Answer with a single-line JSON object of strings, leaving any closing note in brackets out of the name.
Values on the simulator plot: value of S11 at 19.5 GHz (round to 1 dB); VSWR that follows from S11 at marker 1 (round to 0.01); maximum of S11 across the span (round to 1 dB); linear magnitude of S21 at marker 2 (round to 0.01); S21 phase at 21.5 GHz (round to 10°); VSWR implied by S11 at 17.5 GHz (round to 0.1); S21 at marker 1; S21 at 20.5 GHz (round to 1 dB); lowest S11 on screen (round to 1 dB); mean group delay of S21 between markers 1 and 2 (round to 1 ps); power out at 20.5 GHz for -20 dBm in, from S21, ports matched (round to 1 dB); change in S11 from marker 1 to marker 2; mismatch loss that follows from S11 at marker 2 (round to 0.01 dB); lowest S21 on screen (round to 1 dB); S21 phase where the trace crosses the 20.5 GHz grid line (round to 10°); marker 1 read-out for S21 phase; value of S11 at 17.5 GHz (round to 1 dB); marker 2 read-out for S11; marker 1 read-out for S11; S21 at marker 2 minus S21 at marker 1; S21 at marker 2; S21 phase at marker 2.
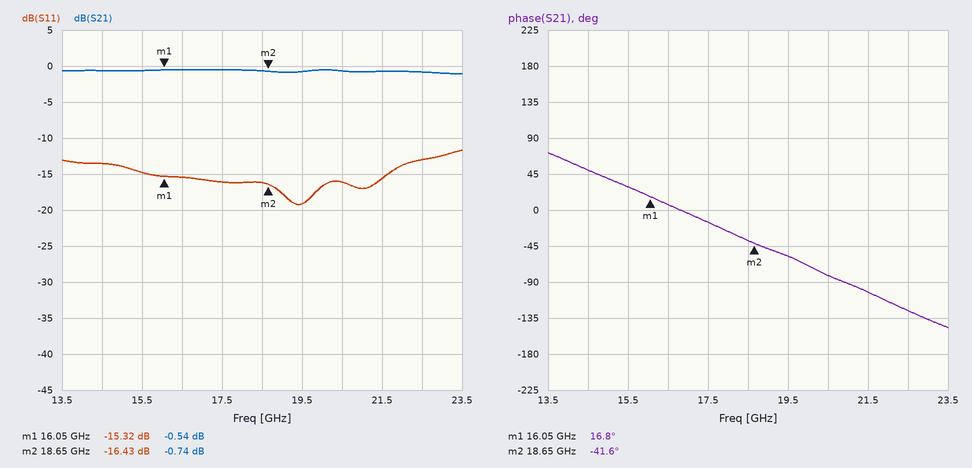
{"value of S11 at 19.5 GHz": "-19 dB", "VSWR that follows from S11 at marker 1": "1.41", "maximum of S11 across the span": "-12 dB", "linear magnitude of S21 at marker 2": "0.92", "S21 phase at 21.5 GHz": "-100°", "VSWR implied by S11 at 17.5 GHz": "1.4", "S21 at marker 1": "-0.54 dB", "S21 at 20.5 GHz": "-1 dB", "lowest S11 on screen": "-19 dB", "mean group delay of S21 between markers 1 and 2": "62 ps", "power out at 20.5 GHz for -20 dBm in, from S21, ports matched": "-21 dBm", "change in S11 from marker 1 to marker 2": "-1.11 dB", "mismatch loss that follows from S11 at marker 2": "0.10 dB", "lowest S21 on screen": "-1 dB", "S21 phase where the trace crosses the 20.5 GHz grid line": "-80°", "marker 1 read-out for S21 phase": "16.8°", "value of S11 at 17.5 GHz": "-16 dB", "marker 2 read-out for S11": "-16.43 dB", "marker 1 read-out for S11": "-15.32 dB", "S21 at marker 2 minus S21 at marker 1": "-0.20 dB", "S21 at marker 2": "-0.74 dB", "S21 phase at marker 2": "-41.6°"}
